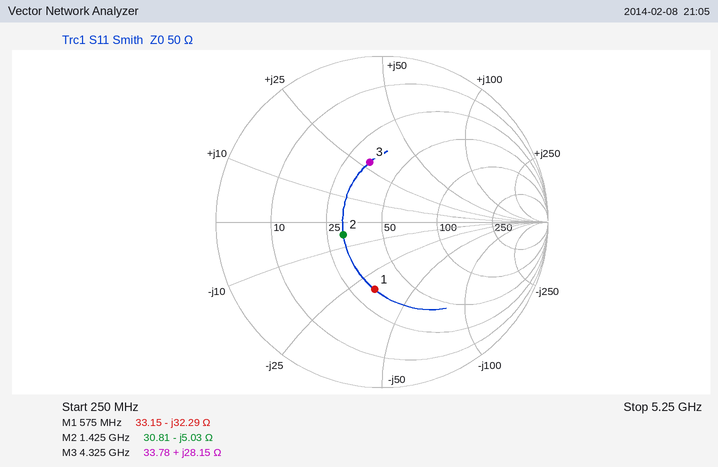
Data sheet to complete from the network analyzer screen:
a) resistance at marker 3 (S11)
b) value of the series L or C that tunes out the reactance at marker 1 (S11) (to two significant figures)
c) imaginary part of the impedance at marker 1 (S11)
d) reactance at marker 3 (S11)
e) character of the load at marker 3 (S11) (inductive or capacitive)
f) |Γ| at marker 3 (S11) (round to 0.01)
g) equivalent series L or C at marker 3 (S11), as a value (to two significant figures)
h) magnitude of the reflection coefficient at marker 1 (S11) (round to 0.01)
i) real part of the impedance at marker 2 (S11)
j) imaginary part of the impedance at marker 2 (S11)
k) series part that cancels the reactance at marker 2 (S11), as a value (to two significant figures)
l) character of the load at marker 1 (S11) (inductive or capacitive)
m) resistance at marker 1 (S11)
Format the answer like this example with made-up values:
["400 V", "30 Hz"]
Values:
["33.78 Ω", "8.9 nH", "-32.29 Ω", "+28.15 Ω", "inductive", "0.37", "1.0 nH", "0.41", "30.81 Ω", "-5.03 Ω", "560 pH", "capacitive", "33.15 Ω"]
